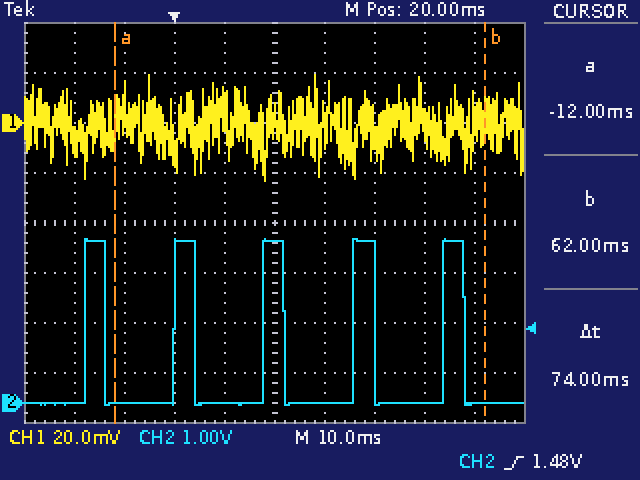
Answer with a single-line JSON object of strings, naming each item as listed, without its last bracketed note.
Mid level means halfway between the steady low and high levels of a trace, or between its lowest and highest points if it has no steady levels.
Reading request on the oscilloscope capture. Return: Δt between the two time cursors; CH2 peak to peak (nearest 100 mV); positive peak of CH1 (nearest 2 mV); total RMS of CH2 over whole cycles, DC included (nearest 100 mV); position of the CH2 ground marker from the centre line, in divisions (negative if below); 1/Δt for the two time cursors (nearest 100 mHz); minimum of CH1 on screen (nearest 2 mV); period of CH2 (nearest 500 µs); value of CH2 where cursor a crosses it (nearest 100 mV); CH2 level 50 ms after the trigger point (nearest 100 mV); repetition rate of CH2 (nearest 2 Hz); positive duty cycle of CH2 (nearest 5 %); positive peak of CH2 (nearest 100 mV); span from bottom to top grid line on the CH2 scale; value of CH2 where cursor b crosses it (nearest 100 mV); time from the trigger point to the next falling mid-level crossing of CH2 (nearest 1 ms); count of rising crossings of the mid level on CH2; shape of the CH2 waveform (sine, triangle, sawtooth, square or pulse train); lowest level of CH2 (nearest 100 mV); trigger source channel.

{"Δt between the two time cursors": "74 ms", "CH2 peak to peak": "3.3 V", "positive peak of CH1": "20 mV", "total RMS of CH2 over whole cycles, DC included": "1.6 V", "position of the CH2 ground marker from the centre line, in divisions": "-3.6 div", "1/Δt for the two time cursors": "13.5 Hz", "minimum of CH1 on screen": "-24 mV", "period of CH2": "18.0 ms", "value of CH2 where cursor a crosses it": "0.0 V", "CH2 level 50 ms after the trigger point": "0.0 V", "repetition rate of CH2": "56 Hz", "positive duty cycle of CH2": "25 %", "positive peak of CH2": "3.3 V", "span from bottom to top grid line on the CH2 scale": "8 V", "value of CH2 where cursor b crosses it": "0.0 V", "time from the trigger point to the next falling mid-level crossing of CH2": "4 ms", "count of rising crossings of the mid level on CH2": "5", "shape of the CH2 waveform": "pulse train", "lowest level of CH2": "0.0 V", "trigger source channel": "CH2"}
